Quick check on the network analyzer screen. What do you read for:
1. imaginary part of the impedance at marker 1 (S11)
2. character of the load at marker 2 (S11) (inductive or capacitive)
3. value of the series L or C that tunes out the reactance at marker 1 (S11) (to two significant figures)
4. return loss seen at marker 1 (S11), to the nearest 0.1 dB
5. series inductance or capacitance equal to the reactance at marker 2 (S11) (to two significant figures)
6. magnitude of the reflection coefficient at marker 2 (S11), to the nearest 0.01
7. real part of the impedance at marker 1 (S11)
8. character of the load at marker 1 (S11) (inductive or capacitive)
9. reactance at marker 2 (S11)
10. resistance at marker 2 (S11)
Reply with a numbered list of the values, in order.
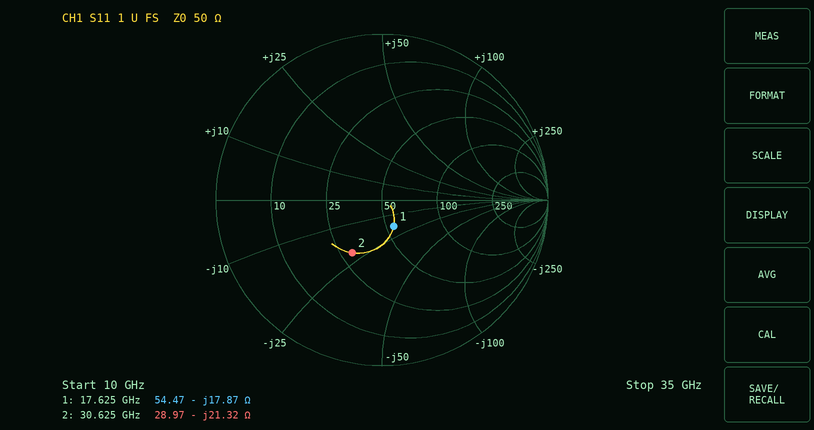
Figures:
1. -17.87 Ω
2. capacitive
3. 160 pH
4. 15.2 dB
5. 240 fF
6. 0.37
7. 54.47 Ω
8. capacitive
9. -21.32 Ω
10. 28.97 Ω
